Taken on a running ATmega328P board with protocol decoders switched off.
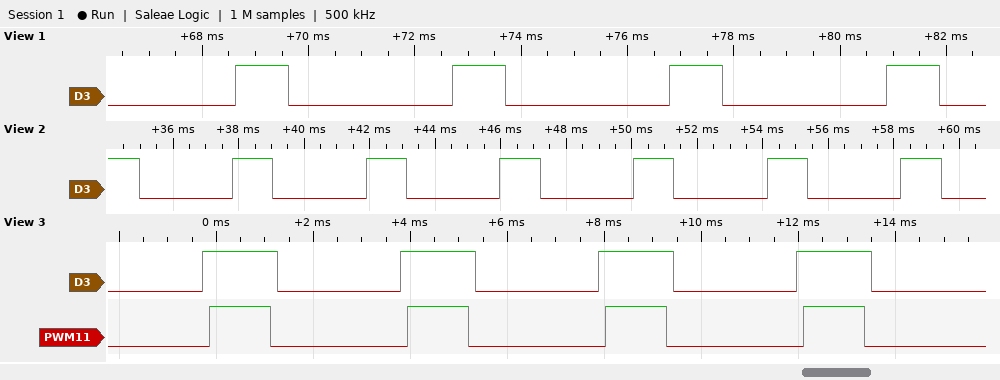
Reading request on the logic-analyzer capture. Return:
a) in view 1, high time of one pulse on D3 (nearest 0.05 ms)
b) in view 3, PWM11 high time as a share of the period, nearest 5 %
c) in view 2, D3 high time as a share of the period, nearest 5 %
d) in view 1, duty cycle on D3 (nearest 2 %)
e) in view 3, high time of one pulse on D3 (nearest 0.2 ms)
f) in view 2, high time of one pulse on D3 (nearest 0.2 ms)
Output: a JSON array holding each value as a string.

["1.00 ms", "30 %", "30 %", "24 %", "1.6 ms", "1.2 ms"]
